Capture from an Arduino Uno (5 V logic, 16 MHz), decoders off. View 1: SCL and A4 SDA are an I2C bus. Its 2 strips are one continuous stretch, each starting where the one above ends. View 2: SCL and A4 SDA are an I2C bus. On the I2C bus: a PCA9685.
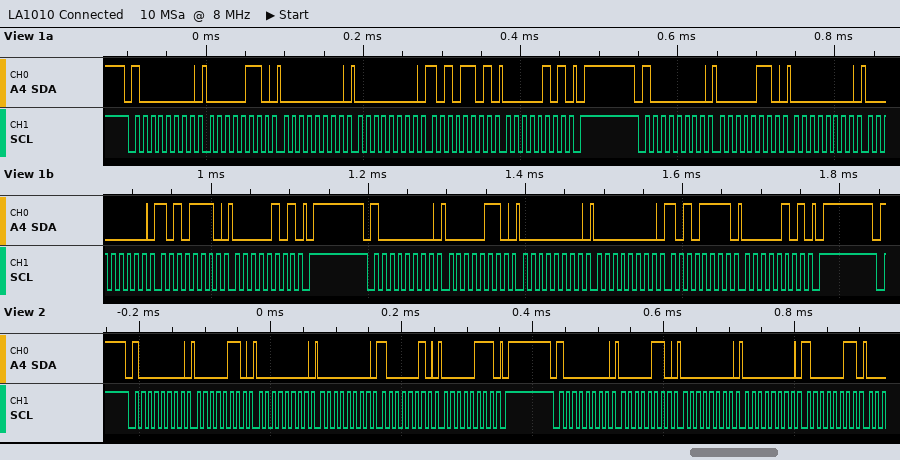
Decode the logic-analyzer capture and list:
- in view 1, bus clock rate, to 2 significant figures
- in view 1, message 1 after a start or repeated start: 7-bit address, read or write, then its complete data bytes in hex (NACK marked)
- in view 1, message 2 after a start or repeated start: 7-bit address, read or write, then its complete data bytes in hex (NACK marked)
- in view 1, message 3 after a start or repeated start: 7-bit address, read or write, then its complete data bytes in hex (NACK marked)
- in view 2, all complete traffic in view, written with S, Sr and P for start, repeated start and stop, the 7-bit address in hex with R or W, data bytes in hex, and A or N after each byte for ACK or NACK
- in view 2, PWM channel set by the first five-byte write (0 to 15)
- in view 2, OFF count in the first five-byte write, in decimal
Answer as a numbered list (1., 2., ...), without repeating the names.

1. 100 kHz
2. 0x40 write: 06 00 00 AD 05
3. 0x40 write: 06 00 00 AE 05
4. 0x40 write: 06 00 00 AF 05
5. S 40W A 06 A 00 A 00 A 82 A 07 A P S 40W A 06 A 00 A 00 A 83 A
6. 0
7. 1922
